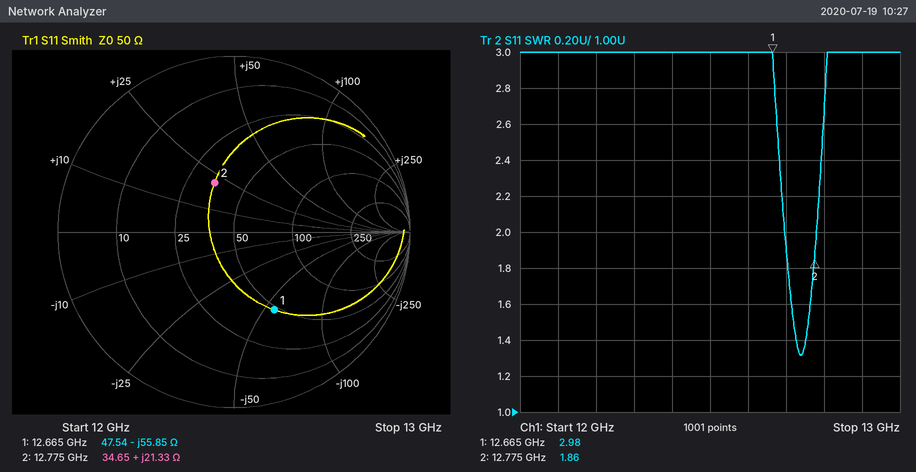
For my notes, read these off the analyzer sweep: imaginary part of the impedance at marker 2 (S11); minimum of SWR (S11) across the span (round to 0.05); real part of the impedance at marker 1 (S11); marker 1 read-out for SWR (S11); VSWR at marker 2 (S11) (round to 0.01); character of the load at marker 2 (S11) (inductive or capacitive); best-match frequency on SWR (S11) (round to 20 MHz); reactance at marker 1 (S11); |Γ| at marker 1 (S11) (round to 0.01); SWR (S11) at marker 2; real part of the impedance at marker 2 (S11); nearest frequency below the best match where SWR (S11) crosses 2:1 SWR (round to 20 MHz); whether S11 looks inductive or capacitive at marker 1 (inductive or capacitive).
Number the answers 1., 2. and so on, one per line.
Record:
1. +21.33 Ω
2. 1.30
3. 47.54 Ω
4. 2.98
5. 1.86
6. inductive
7. 12.74 GHz
8. -55.85 Ω
9. 0.50
10. 1.86
11. 34.65 Ω
12. 12.70 GHz
13. capacitive
